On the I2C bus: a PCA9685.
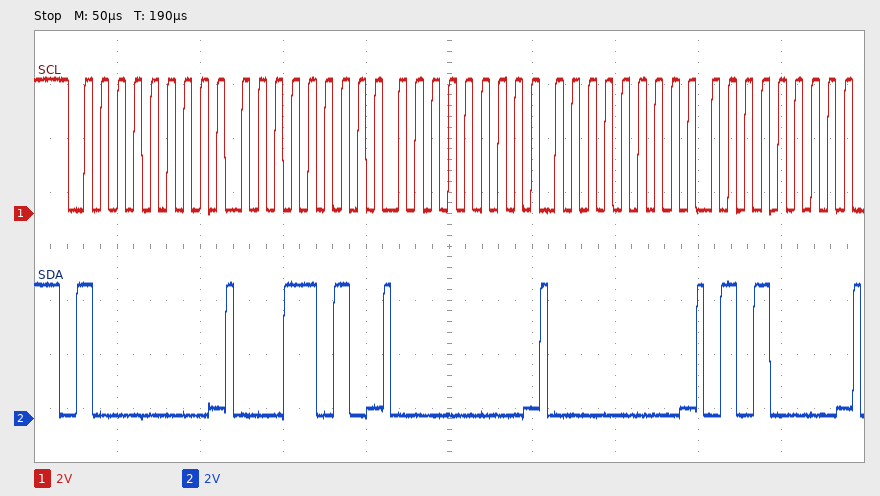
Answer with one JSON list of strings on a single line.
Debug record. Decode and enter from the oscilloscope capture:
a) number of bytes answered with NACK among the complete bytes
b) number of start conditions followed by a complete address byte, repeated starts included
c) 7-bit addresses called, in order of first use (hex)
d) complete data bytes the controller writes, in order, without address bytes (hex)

["0", "1", "0x40", "1A 00 00 50"]
